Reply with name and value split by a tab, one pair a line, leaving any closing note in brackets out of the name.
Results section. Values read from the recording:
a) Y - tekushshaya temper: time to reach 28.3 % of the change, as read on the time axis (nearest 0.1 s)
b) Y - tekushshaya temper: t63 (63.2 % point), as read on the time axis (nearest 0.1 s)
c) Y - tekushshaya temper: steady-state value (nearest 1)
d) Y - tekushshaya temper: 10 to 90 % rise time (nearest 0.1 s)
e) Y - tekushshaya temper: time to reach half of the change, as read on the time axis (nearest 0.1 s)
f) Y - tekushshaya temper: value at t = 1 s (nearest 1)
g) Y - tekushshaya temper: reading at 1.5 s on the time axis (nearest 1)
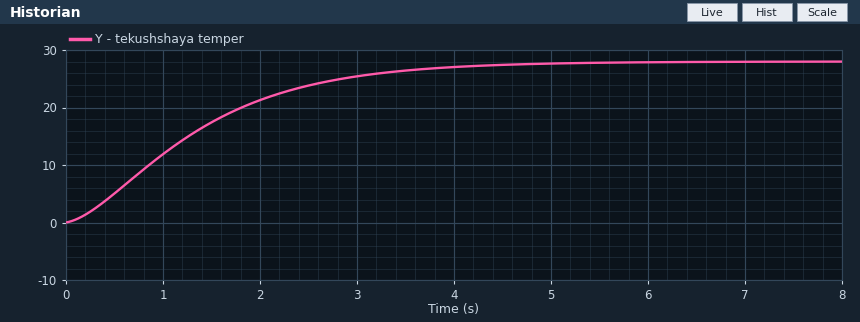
Y - tekushshaya temper: time to reach 28.3 % of the change, as read on the time axis	0.7 s
Y - tekushshaya temper: t63 (63.2 % point), as read on the time axis	1.5 s
Y - tekushshaya temper: steady-state value	28
Y - tekushshaya temper: 10 to 90 % rise time	2.6 s
Y - tekushshaya temper: time to reach half of the change, as read on the time axis	1.2 s
Y - tekushshaya temper: value at t = 1 s	12
Y - tekushshaya temper: reading at 1.5 s on the time axis	17
